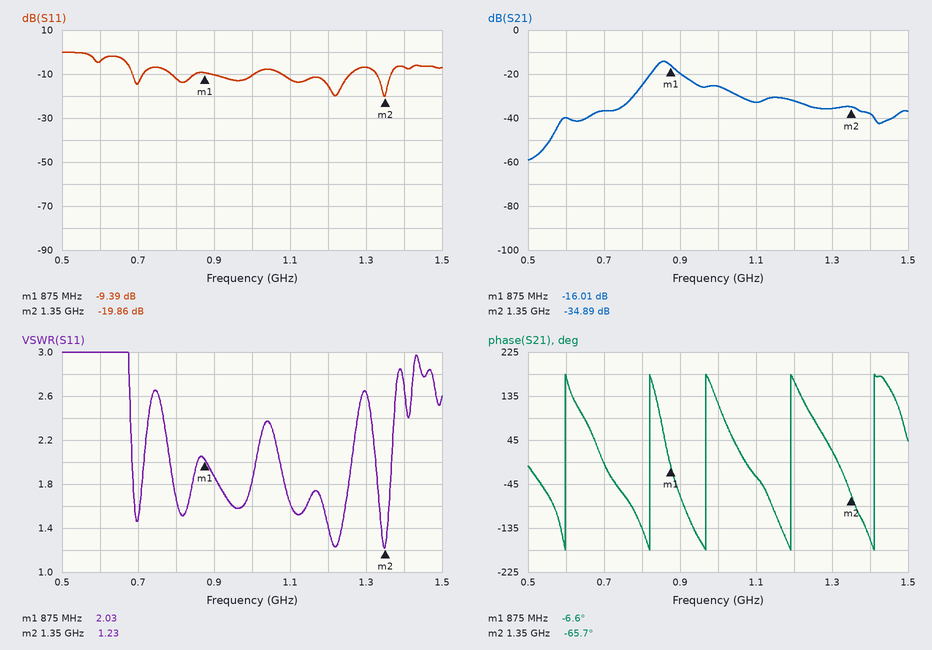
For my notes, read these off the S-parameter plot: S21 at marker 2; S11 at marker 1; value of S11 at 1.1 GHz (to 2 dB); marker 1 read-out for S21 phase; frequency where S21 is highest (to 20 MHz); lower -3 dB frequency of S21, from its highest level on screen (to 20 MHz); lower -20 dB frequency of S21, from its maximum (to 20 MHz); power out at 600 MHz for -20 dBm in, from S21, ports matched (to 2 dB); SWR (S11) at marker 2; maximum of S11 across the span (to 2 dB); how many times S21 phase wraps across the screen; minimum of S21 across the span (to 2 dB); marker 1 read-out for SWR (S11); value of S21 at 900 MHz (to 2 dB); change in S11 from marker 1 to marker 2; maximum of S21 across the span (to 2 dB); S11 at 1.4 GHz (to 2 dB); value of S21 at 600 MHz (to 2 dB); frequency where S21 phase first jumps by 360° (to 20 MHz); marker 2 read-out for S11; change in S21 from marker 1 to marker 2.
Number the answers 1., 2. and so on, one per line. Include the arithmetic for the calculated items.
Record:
1. -34.89 dB
2. -9.39 dB
3. -12 dB
4. -6.6°
5. 860 MHz
6. 840 MHz
7. 760 MHz
8. -20 dBm + (-40 dB) = -60 dBm
9. 1.23
10. 0 dB
11. 5
12. -60 dB
13. 2.03
14. -20 dB
15. -19.86 − (-9.39) = -10.47 dB
16. -14 dB
17. -6 dB
18. -40 dB
19. 600 MHz
20. -19.86 dB
21. -34.89 − (-16.01) = -18.88 dB
